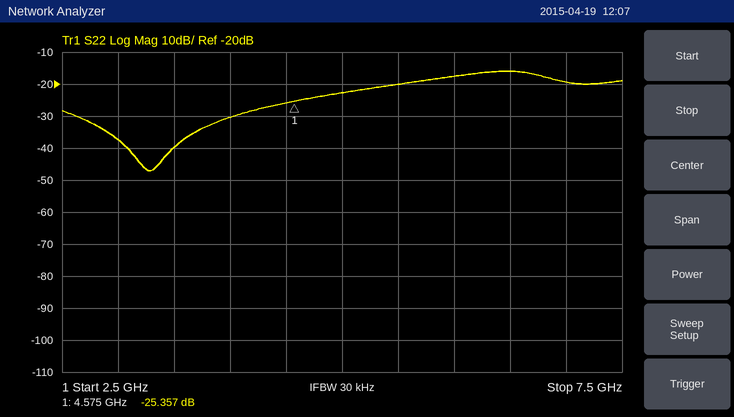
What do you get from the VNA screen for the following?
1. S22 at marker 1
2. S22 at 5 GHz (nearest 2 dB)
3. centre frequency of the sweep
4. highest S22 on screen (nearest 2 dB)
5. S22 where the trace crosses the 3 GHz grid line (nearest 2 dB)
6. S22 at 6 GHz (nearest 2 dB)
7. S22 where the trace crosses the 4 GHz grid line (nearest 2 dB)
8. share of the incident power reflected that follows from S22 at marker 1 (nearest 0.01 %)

-25.357 dB
-22 dB
5 GHz
-16 dB
-38 dB
-18 dB
-30 dB
0.29 %
